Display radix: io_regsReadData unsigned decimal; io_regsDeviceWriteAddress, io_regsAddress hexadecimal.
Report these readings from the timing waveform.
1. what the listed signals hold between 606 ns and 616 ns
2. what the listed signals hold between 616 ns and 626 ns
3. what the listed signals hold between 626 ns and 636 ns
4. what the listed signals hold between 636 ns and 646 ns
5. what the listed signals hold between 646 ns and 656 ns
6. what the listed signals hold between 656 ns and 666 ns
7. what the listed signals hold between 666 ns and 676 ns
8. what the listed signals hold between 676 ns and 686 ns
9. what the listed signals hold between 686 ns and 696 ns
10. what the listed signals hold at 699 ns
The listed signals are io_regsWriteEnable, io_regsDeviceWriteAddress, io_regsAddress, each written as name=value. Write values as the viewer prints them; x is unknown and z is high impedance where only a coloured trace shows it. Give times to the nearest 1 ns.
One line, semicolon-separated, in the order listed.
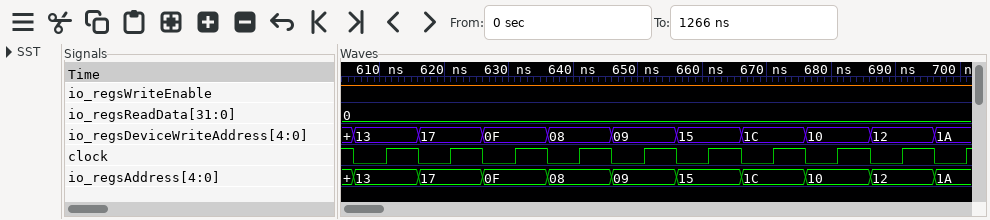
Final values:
io_regsWriteEnable=1, io_regsDeviceWriteAddress=13, io_regsAddress=13; io_regsWriteEnable=1, io_regsDeviceWriteAddress=17, io_regsAddress=17; io_regsWriteEnable=1, io_regsDeviceWriteAddress=0F, io_regsAddress=0F; io_regsWriteEnable=1, io_regsDeviceWriteAddress=08, io_regsAddress=08; io_regsWriteEnable=1, io_regsDeviceWriteAddress=09, io_regsAddress=09; io_regsWriteEnable=1, io_regsDeviceWriteAddress=15, io_regsAddress=15; io_regsWriteEnable=1, io_regsDeviceWriteAddress=1C, io_regsAddress=1C; io_regsWriteEnable=1, io_regsDeviceWriteAddress=10, io_regsAddress=10; io_regsWriteEnable=1, io_regsDeviceWriteAddress=12, io_regsAddress=12; io_regsWriteEnable=1, io_regsDeviceWriteAddress=1A, io_regsAddress=1A
